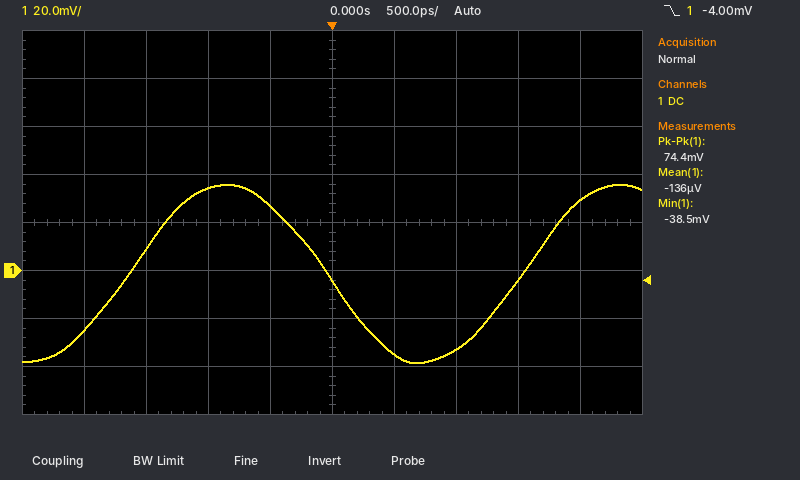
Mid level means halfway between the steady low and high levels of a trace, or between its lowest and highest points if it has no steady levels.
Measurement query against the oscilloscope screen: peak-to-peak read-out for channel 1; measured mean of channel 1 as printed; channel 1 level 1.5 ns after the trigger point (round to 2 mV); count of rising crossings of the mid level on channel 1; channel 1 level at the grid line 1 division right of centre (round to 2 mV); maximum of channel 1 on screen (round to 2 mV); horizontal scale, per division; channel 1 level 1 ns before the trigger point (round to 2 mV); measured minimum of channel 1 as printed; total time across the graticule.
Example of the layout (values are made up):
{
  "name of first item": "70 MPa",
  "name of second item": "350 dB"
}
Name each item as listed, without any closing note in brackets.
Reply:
{
  "peak-to-peak read-out for channel 1": "74.4 mV",
  "measured mean of channel 1 as printed": "-136 µV",
  "channel 1 level 1.5 ns after the trigger point": "-4 mV",
  "count of rising crossings of the mid level on channel 1": "2",
  "channel 1 level at the grid line 1 division right of centre": "-34 mV",
  "maximum of channel 1 on screen": "36 mV",
  "horizontal scale, per division": "500 ps",
  "channel 1 level 1 ns before the trigger point": "34 mV",
  "measured minimum of channel 1 as printed": "-38.5 mV",
  "total time across the graticule": "5 ns"
}
